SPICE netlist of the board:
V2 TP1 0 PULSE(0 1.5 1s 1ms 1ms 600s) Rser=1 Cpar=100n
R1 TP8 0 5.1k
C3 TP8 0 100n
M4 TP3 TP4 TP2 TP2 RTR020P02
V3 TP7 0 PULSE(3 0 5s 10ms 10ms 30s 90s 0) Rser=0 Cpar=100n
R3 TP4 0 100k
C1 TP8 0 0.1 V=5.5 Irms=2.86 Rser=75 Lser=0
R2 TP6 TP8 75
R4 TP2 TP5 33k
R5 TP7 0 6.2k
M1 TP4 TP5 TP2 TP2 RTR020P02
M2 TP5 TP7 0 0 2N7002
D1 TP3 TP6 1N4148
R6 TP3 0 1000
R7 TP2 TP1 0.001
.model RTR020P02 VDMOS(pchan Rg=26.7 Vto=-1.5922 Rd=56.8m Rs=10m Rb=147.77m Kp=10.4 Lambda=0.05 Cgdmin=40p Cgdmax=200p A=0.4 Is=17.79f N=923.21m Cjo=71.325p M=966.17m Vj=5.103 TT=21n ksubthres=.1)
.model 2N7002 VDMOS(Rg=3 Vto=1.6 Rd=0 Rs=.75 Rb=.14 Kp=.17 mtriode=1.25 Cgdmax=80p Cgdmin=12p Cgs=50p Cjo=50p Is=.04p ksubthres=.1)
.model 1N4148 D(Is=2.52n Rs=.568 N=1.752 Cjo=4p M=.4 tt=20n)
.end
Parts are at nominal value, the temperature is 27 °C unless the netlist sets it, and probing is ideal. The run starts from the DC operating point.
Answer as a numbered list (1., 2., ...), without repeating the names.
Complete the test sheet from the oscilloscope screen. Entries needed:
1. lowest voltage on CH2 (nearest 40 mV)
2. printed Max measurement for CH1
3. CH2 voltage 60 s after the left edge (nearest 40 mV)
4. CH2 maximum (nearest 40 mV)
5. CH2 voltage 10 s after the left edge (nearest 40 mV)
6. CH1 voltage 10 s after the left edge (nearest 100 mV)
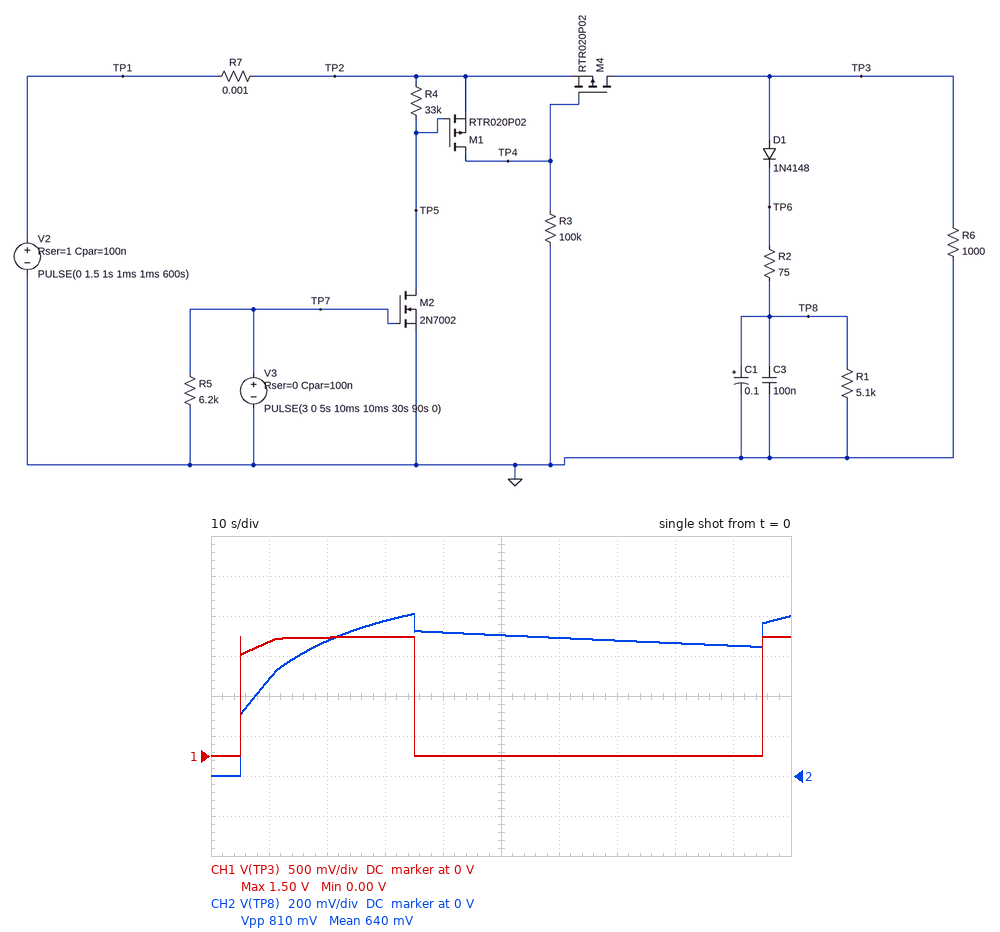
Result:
1. 0 V
2. 1.50 V
3. 680 mV
4. 800 mV
5. 480 mV
6. 1.4 V
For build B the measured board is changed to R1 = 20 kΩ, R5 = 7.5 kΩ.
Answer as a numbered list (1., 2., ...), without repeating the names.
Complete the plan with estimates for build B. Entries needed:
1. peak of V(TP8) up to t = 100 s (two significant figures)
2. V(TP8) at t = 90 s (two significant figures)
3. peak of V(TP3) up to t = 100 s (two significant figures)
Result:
1. 840 mV
2. 720 mV
3. 1.5 V
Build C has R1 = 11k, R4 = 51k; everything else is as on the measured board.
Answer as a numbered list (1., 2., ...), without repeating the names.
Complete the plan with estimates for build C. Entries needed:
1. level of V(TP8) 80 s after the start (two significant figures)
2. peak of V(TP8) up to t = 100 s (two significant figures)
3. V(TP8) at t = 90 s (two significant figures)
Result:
1. 710 mV
2. 830 mV
3. 700 mV
